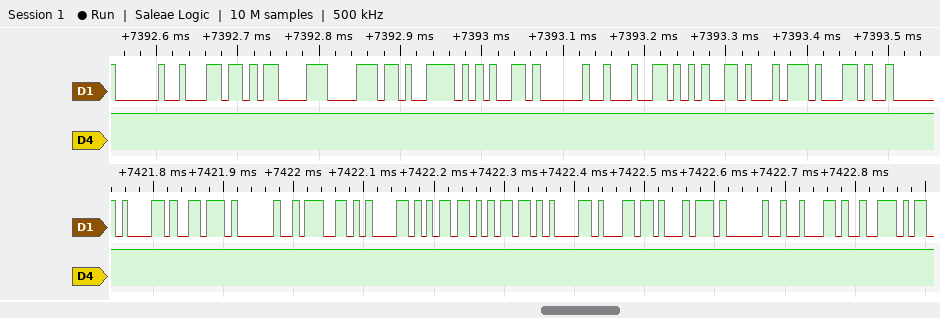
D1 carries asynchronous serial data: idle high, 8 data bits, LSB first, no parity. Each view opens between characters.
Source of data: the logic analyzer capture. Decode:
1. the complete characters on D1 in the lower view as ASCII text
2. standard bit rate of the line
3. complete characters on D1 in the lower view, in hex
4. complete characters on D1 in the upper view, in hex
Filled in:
"av gammalt br"
115200 baud
61, 76, 20, 67, 61, 6D, 6D, 61, 6C, 74, 20, 62, 72
20, 6C, C3, B8, 79, 65, 20, 64, 65, 74, 2C
